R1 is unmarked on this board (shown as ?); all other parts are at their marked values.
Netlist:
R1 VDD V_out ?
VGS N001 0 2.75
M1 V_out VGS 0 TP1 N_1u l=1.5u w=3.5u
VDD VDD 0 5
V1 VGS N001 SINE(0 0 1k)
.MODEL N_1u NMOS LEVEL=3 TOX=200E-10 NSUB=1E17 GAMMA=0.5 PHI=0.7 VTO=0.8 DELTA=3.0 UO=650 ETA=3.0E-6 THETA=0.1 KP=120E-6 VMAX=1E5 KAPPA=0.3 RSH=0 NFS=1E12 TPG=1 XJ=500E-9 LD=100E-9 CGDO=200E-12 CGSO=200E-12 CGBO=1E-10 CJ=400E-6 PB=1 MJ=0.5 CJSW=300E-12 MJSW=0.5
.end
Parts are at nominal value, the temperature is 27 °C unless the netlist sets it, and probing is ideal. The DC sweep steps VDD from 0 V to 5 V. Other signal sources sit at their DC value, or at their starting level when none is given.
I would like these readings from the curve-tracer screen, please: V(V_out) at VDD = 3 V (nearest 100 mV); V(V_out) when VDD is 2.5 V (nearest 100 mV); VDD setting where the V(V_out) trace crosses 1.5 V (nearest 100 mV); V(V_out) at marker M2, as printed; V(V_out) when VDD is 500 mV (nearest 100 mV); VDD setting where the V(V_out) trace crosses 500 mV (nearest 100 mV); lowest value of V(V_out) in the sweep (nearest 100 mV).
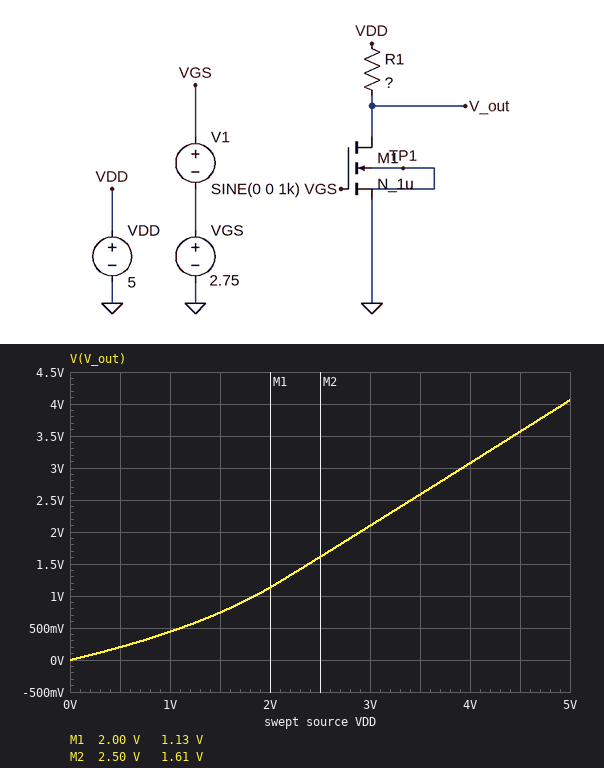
2.1 V
1.6 V
2.4 V
1.61 V
200 mV
1.1 V
0 V
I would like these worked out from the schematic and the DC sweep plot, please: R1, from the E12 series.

3.3 kΩ
